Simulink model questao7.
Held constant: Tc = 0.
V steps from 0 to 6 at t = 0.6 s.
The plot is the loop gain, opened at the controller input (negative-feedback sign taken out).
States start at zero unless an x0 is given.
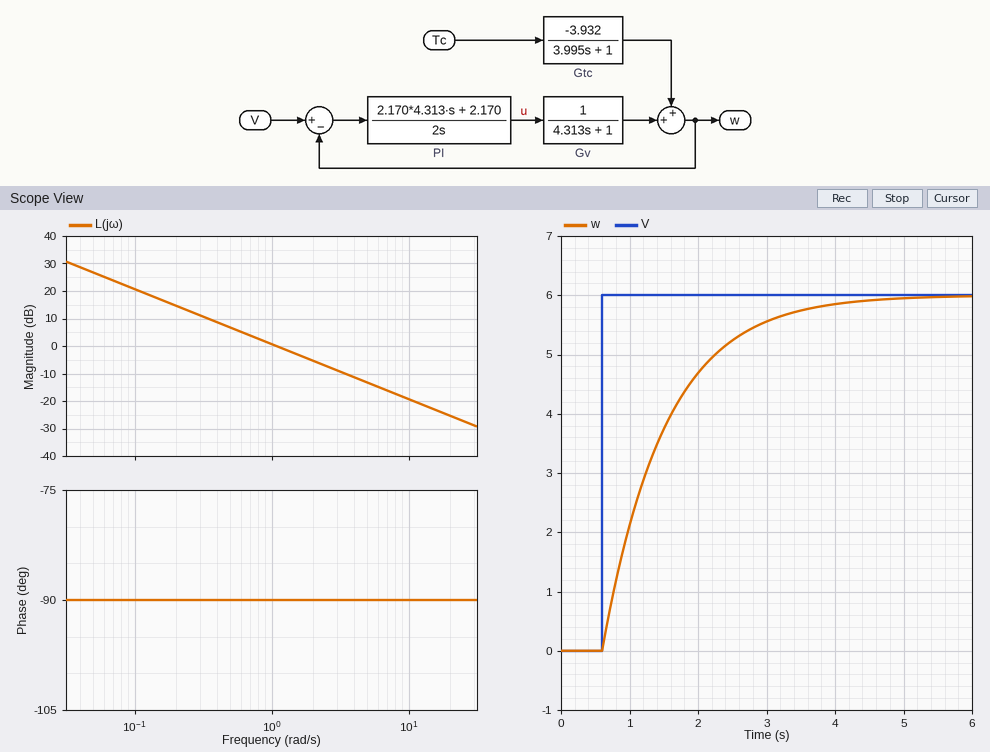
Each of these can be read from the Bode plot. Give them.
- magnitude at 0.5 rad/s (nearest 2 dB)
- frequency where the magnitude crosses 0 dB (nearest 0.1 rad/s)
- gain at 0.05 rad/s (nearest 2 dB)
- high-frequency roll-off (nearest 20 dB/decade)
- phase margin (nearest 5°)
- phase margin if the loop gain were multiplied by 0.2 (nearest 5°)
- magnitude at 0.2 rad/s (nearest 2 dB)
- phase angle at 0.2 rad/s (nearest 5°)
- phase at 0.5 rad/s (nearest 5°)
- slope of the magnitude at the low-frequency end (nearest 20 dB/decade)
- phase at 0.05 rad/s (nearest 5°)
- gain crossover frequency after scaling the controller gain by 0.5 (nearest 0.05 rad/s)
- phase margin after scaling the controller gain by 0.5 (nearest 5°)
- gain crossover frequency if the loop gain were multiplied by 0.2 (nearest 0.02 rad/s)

6 dB
1.1 rad/s
26 dB
-20 dB/decade
90°
90°
14 dB
-90°
-90°
-20 dB/decade
-90°
0.55 rad/s
90°
0.22 rad/s
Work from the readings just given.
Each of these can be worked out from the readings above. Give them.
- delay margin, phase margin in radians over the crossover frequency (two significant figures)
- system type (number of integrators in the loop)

1.4 s
1
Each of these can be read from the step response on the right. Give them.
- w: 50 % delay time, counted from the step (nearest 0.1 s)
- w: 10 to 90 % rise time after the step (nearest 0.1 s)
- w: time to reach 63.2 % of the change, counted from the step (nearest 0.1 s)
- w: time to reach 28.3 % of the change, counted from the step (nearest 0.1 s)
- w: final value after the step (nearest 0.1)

0.6 s
2.0 s
0.9 s
0.3 s
6.0
